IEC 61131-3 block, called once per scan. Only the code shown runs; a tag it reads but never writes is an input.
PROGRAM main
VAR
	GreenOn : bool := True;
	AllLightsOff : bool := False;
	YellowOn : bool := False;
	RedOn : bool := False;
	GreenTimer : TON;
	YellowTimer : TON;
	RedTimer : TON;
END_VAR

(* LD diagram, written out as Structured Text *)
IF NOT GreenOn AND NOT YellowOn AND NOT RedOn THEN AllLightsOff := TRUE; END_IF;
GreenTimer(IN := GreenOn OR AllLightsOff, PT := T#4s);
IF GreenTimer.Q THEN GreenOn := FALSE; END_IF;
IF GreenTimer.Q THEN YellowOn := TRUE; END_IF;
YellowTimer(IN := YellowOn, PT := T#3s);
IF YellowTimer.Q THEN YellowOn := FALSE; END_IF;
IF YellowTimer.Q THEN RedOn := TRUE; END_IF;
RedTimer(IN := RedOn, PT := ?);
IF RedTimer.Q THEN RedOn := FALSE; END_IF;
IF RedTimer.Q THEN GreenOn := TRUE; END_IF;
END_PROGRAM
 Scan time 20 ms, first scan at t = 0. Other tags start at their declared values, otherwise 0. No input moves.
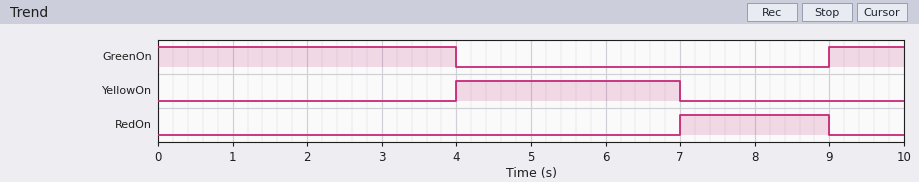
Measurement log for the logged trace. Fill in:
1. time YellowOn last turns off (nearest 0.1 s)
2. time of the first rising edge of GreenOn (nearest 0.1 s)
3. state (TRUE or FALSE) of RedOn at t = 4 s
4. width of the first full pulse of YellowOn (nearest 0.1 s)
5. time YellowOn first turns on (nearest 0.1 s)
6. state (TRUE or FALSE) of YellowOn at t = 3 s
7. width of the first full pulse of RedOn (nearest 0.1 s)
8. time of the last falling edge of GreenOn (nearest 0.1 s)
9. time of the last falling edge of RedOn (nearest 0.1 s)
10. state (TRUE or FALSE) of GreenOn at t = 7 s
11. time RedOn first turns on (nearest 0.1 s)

7.0 s
9.0 s
FALSE
3.0 s
4.0 s
FALSE
2.0 s
4.0 s
9.0 s
FALSE
7.0 s
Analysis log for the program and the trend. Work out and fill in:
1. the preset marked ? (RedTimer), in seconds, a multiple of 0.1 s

2.0 s
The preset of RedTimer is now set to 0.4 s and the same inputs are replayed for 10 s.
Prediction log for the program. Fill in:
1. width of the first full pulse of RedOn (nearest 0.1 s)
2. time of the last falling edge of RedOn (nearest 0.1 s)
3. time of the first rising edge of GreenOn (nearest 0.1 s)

0.4 s
7.4 s
7.4 s
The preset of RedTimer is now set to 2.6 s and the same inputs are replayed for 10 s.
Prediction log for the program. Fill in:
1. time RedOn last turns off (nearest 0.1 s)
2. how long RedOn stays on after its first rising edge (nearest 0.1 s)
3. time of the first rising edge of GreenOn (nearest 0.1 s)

9.6 s
2.6 s
9.6 s
